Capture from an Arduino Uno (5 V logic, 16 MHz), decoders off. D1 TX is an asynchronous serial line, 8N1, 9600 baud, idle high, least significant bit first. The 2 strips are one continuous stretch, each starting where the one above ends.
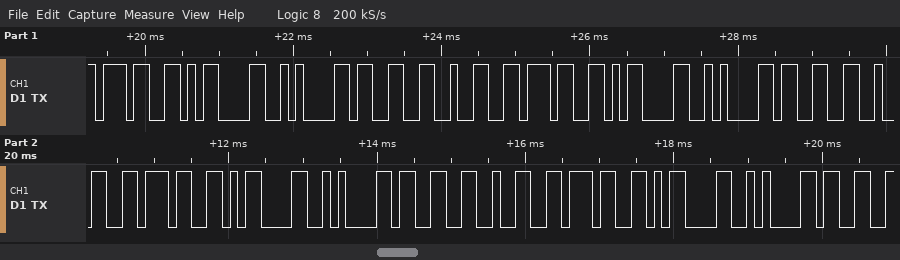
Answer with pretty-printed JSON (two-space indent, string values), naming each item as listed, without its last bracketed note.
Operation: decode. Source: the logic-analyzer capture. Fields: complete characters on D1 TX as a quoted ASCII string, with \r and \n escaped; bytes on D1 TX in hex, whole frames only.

{
  "complete characters on D1 TX as a quoted ASCII string, with \\r and \\n escaped": "\"7\\r\\n327\\r\\n327\\r\\n327\\r\\n3\"",
  "bytes on D1 TX in hex, whole frames only": "37 0D 0A 33 32 37 0D 0A 33 32 37 0D 0A 33 32 37 0D 0A 33"
}
